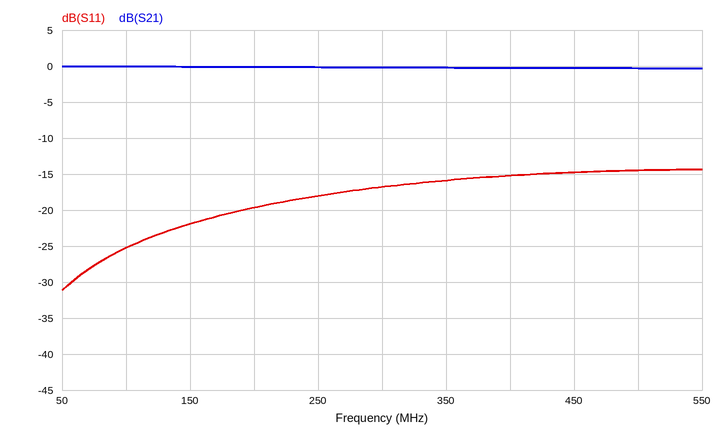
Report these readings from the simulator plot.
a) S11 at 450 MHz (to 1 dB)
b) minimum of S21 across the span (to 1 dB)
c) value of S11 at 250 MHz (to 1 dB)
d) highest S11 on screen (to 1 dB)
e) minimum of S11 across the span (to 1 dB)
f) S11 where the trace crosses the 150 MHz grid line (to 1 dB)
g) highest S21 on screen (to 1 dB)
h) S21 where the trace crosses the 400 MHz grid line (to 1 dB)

-15 dB
0 dB
-18 dB
-14 dB
-31 dB
-22 dB
0 dB
0 dB
